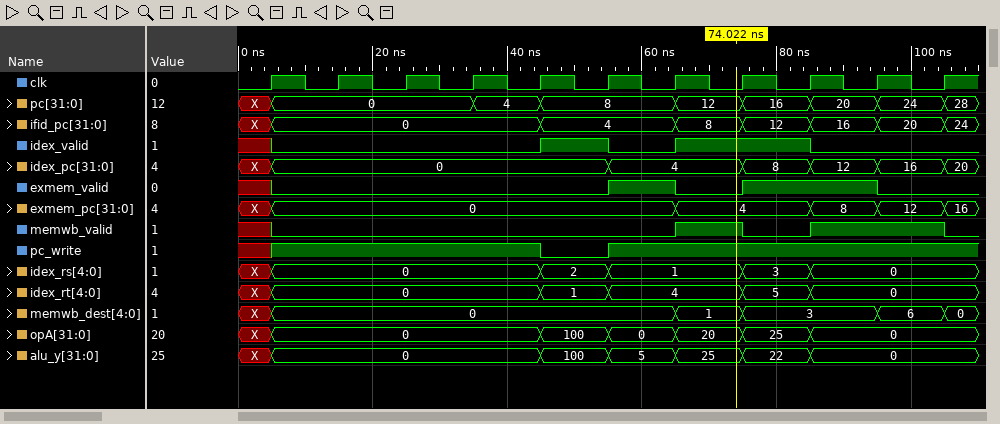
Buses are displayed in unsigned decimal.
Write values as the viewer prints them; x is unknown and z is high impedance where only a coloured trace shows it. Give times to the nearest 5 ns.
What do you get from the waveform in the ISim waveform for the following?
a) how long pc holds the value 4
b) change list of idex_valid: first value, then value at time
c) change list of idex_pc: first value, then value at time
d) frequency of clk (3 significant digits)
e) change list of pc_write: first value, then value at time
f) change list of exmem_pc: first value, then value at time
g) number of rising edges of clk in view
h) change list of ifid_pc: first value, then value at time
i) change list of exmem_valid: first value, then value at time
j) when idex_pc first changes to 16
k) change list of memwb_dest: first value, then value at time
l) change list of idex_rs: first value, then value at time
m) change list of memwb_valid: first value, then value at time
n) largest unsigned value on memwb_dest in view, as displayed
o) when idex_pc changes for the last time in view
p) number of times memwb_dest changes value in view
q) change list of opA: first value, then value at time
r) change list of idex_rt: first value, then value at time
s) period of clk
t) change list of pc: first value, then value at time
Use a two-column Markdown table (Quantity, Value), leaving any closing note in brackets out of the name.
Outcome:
| Quantity | Value |
|---|---|
| how long pc holds the value 4 | 10 ns |
| change list of idex_valid: first value, then value at time | x, 0 at 5 ns, 1 at 45 ns, 0 at 55 ns, 1 at 65 ns, 0 at 85 ns |
| change list of idex_pc: first value, then value at time | X, 0 at 5 ns, 4 at 55 ns, 8 at 75 ns, 12 at 85 ns, 16 at 95 ns, 20 at 105 ns |
| frequency of clk | 100 MHz |
| change list of pc_write: first value, then value at time | x, 1 at 5 ns, 0 at 45 ns, 1 at 55 ns |
| change list of exmem_pc: first value, then value at time | X, 0 at 5 ns, 4 at 65 ns, 8 at 85 ns, 12 at 95 ns, 16 at 105 ns |
| number of rising edges of clk in view | 11 |
| change list of ifid_pc: first value, then value at time | X, 0 at 5 ns, 4 at 45 ns, 8 at 65 ns, 12 at 75 ns, 16 at 85 ns, 20 at 95 ns, 24 at 105 ns |
| change list of exmem_valid: first value, then value at time | x, 0 at 5 ns, 1 at 55 ns, 0 at 65 ns, 1 at 75 ns, 0 at 95 ns |
| when idex_pc first changes to 16 | 95 ns |
| change list of memwb_dest: first value, then value at time | X, 0 at 5 ns, 1 at 65 ns, 3 at 75 ns, 6 at 95 ns, 0 at 105 ns |
| change list of idex_rs: first value, then value at time | X, 0 at 5 ns, 2 at 45 ns, 1 at 55 ns, 3 at 75 ns, 0 at 85 ns |
| change list of memwb_valid: first value, then value at time | x, 0 at 5 ns, 1 at 65 ns, 0 at 75 ns, 1 at 85 ns, 0 at 105 ns |
| largest unsigned value on memwb_dest in view, as displayed | 6 |
| when idex_pc changes for the last time in view | 105 ns |
| number of times memwb_dest changes value in view | 5 |
| change list of opA: first value, then value at time | X, 0 at 5 ns, 100 at 45 ns, 0 at 55 ns, 20 at 65 ns, 25 at 75 ns, 0 at 85 ns |
| change list of idex_rt: first value, then value at time | X, 0 at 5 ns, 1 at 45 ns, 4 at 55 ns, 5 at 75 ns, 0 at 85 ns |
| period of clk | 10 ns |
| change list of pc: first value, then value at time | X, 0 at 5 ns, 4 at 35 ns, 8 at 45 ns, 12 at 65 ns, 16 at 75 ns, 20 at 85 ns, 24 at 95 ns, 28 at 105 ns |
